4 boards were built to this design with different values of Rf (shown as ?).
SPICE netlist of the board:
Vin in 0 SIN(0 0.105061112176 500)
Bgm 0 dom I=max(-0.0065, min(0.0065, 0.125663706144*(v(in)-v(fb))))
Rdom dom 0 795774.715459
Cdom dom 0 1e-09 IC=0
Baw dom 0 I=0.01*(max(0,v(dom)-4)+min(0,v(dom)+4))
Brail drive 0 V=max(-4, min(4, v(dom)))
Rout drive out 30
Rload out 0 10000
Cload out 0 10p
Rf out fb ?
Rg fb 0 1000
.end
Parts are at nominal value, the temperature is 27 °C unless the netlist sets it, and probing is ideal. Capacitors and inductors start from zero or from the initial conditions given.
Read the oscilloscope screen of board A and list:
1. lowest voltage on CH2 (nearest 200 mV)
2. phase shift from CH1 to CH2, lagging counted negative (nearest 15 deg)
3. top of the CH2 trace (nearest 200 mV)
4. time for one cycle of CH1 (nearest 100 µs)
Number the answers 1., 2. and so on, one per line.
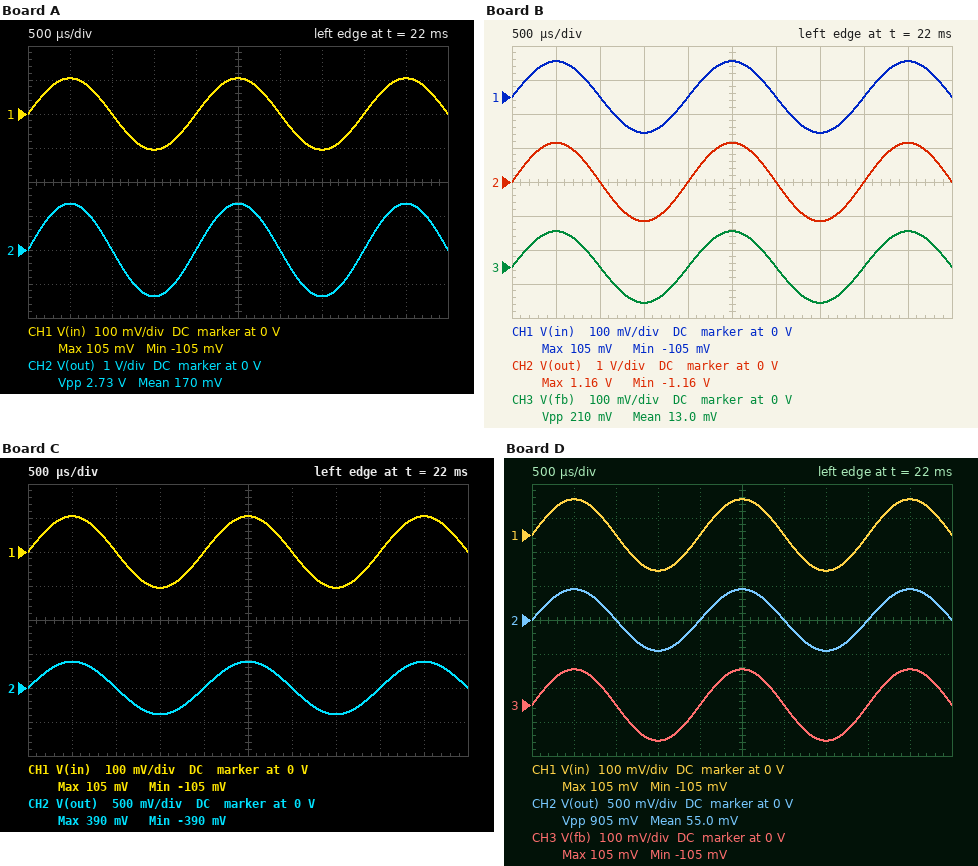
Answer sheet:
1. -1.4 V
2. 0 deg
3. 1.4 V
4. 2.0 ms
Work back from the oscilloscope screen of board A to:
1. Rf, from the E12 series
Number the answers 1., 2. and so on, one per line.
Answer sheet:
1. 12 kΩ
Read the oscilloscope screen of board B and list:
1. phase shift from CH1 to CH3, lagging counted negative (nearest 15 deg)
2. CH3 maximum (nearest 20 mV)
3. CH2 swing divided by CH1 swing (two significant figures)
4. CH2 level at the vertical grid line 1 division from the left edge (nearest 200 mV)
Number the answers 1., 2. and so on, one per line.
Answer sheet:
1. 0 deg
2. 100 mV
3. 11
4. 1.2 V
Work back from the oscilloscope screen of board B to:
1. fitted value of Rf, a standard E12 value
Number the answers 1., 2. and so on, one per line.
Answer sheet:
1. 10 kΩ
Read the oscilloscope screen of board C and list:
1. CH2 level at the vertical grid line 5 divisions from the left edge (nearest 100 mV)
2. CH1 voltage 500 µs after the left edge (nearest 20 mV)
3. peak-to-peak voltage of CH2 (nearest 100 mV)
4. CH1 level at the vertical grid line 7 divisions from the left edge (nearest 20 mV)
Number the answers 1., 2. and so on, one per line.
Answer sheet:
1. 400 mV
2. 100 mV
3. 800 mV
4. -100 mV
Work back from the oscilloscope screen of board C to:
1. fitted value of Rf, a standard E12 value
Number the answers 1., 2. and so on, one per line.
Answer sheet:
1. 2.7 kΩ
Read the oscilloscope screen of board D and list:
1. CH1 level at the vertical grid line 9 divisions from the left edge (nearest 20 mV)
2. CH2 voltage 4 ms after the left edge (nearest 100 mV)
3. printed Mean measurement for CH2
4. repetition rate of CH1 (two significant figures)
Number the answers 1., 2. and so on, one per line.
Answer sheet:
1. 100 mV
2. 0 V
3. 55.0 mV
4. 500 Hz
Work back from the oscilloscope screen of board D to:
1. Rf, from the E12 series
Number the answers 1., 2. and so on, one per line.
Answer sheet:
1. 3.3 kΩ
